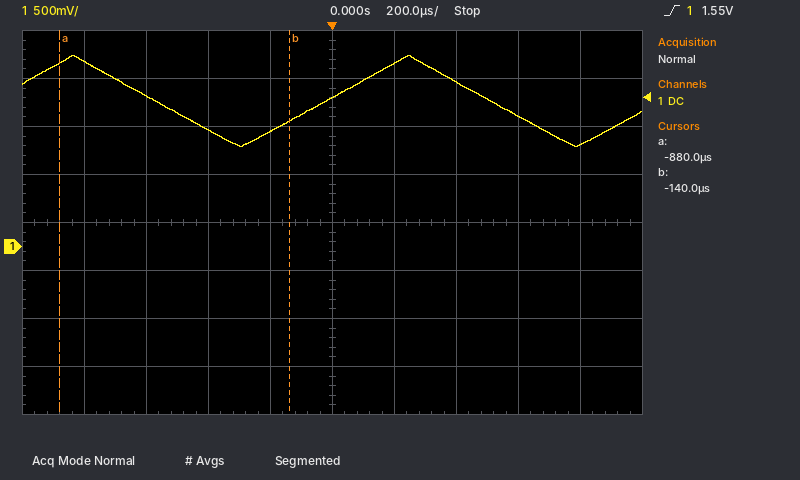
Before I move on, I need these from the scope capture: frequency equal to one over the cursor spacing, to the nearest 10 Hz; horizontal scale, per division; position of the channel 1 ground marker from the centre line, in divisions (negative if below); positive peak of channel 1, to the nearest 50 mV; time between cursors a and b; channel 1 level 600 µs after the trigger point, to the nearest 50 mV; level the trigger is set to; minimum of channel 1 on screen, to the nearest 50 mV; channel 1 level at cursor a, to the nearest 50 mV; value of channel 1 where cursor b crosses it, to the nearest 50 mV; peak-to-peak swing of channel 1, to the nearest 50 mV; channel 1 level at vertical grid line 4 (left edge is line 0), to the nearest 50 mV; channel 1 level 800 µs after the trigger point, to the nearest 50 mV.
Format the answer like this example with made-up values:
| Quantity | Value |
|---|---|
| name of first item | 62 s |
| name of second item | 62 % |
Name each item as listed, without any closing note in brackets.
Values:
| Quantity | Value |
|---|---|
| frequency equal to one over the cursor spacing, to the nearest 10 Hz | 1.35 kHz |
| horizontal scale, per division | 200 µs |
| position of the channel 1 ground marker from the centre line, in divisions | -0.5 div |
| positive peak of channel 1, to the nearest 50 mV | 2.00 V |
| time between cursors a and b | 740 µs |
| channel 1 level 600 µs after the trigger point, to the nearest 50 mV | 1.35 V |
| level the trigger is set to | 1.55 V |
| minimum of channel 1 on screen, to the nearest 50 mV | 1.05 V |
| channel 1 level at cursor a, to the nearest 50 mV | 1.90 V |
| value of channel 1 where cursor b crosses it, to the nearest 50 mV | 1.30 V |
| peak-to-peak swing of channel 1, to the nearest 50 mV | 950 mV |
| channel 1 level at vertical grid line 4 (left edge is line 0), to the nearest 50 mV | 1.20 V |
| channel 1 level 800 µs after the trigger point, to the nearest 50 mV | 1.05 V |
